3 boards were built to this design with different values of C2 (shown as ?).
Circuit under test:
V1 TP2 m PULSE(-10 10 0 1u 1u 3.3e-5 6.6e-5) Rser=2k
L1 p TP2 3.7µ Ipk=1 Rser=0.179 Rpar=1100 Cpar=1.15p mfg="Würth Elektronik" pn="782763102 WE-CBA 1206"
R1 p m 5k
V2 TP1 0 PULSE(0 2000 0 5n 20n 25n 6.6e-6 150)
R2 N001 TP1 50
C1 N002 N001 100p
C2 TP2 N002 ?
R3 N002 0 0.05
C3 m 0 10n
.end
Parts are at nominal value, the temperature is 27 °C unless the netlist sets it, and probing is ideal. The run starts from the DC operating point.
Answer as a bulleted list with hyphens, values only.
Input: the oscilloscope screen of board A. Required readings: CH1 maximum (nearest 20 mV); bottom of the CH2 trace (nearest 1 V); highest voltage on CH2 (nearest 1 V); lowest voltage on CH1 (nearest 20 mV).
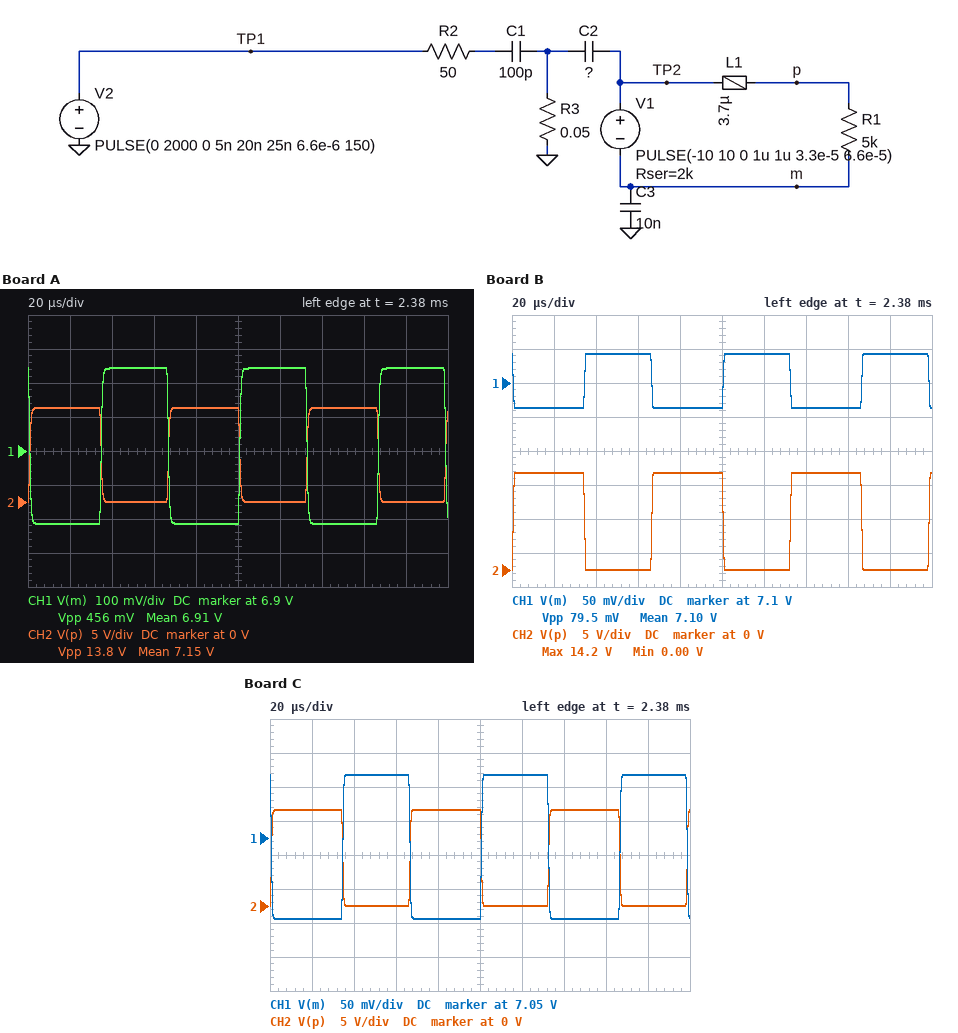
- 7.14 V
- 0 V
- 14 V
- 6.68 V
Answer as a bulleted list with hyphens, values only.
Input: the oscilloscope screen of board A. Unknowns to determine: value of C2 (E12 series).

- 330 pF
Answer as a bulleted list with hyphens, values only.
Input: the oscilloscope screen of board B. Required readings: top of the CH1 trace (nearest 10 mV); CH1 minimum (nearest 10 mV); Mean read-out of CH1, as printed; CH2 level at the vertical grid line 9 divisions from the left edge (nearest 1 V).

- 7.14 V
- 7.06 V
- 7.10 V
- 0 V
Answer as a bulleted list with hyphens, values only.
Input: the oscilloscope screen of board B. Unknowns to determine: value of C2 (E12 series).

- 56 pF
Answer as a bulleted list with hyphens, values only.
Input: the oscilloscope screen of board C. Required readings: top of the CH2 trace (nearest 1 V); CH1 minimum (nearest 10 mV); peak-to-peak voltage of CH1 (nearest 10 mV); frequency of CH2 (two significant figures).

- 14 V
- 6.93 V
- 210 mV
- 15 kHz
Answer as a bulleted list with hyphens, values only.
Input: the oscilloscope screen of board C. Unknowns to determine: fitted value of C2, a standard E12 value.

- 150 pF
